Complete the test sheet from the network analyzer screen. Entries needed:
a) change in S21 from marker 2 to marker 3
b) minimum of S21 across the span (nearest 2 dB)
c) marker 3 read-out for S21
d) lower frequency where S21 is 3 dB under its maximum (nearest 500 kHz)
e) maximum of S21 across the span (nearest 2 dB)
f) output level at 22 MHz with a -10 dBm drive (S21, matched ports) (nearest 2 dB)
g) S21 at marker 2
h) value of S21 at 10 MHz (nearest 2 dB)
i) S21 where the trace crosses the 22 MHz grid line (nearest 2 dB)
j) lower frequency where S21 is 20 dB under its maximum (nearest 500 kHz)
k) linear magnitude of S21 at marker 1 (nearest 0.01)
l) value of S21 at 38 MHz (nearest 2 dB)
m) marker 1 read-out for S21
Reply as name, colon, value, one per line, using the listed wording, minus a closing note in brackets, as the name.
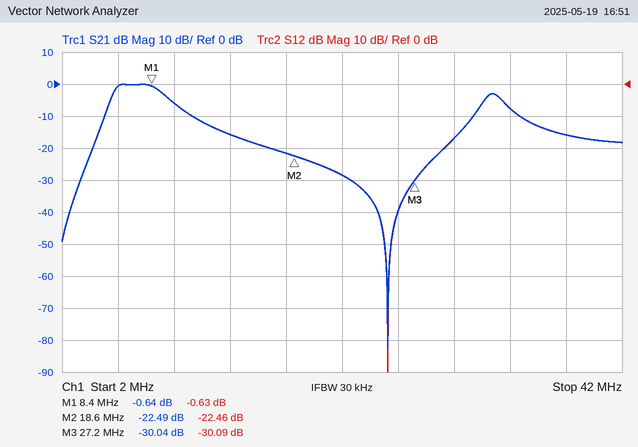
change in S21 from marker 2 to marker 3: -7.55 dB
minimum of S21 across the span: -82 dB
marker 3 read-out for S21: -30.04 dB
lower frequency where S21 is 3 dB under its maximum: 5.5 MHz
maximum of S21 across the span: 0 dB
output level at 22 MHz with a -10 dBm drive (S21, matched ports): -38 dBm
S21 at marker 2: -22.49 dB
value of S21 at 10 MHz: -6 dB
S21 where the trace crosses the 22 MHz grid line: -28 dB
lower frequency where S21 is 20 dB under its maximum: 4.0 MHz
linear magnitude of S21 at marker 1: 0.93
value of S21 at 38 MHz: -16 dB
marker 1 read-out for S21: -0.64 dB
